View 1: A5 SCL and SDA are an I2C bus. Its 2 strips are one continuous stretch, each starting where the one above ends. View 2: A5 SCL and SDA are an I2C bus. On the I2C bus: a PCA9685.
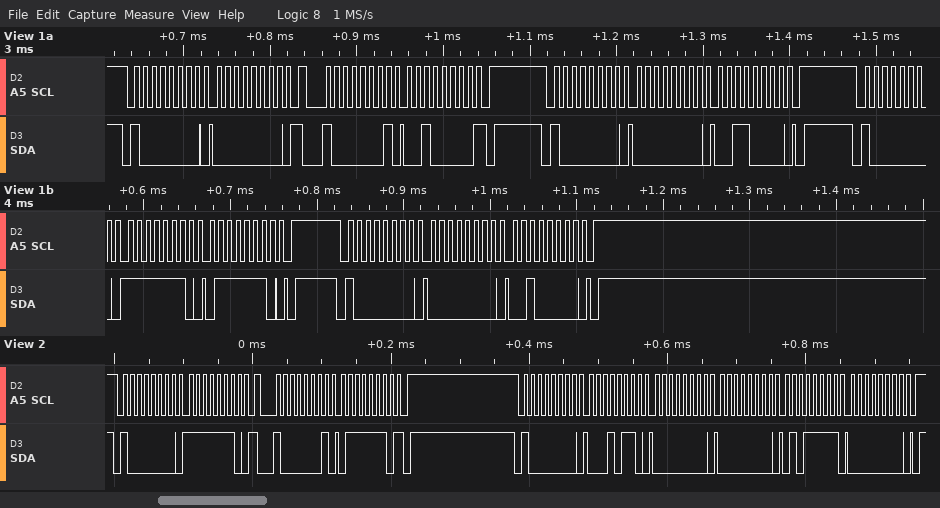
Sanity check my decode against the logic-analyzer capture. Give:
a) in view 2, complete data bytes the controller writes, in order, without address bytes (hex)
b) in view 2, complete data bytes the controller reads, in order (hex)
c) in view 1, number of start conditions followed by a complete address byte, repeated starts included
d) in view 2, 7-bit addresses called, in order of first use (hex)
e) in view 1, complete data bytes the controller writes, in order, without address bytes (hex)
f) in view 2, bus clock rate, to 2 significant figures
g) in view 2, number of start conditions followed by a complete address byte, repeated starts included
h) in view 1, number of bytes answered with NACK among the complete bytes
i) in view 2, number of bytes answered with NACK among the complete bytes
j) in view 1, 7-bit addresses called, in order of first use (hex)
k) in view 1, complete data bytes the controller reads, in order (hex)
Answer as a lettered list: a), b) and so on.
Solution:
a) FE 16 00 00 5F 00
b) 7E
c) 5
d) 0x40
e) 00 00 30 FE 7E 00 20
f) 100 kHz
g) 3
h) 1
i) 1
j) 0x40
k) 20
